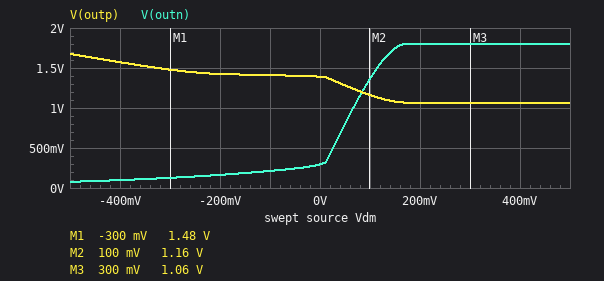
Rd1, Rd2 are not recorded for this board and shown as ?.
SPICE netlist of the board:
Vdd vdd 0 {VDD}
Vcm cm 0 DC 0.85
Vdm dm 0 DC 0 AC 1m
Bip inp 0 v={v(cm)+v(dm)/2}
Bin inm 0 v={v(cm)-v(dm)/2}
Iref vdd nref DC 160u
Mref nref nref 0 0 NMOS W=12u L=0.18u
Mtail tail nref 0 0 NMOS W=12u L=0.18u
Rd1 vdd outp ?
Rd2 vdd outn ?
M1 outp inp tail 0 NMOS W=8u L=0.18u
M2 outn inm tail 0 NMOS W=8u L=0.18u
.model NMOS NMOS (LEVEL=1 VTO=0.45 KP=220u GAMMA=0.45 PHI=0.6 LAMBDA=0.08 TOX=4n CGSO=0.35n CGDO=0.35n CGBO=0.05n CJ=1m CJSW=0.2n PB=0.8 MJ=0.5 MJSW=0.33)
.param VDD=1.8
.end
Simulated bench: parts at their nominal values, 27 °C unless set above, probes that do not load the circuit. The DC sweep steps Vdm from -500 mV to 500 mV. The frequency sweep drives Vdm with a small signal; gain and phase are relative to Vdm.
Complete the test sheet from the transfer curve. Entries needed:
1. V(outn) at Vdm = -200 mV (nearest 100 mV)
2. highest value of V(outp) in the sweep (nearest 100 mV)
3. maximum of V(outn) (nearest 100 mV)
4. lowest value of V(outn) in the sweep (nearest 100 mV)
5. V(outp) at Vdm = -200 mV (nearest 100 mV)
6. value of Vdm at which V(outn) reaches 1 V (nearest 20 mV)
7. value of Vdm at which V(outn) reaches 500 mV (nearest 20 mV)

200 mV
1.7 V
1.8 V
100 mV
1.4 V
60 mV
20 mV
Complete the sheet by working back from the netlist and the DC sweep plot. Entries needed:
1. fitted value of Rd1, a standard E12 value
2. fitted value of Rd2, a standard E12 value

4.7 kΩ
22 kΩ
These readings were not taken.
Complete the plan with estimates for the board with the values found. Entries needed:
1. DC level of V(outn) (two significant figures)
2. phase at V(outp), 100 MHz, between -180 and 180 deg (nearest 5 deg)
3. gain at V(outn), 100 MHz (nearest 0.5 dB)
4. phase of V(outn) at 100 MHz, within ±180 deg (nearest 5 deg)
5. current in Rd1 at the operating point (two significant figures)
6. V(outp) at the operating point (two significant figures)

290 mV
-170 deg
4.5 dB
0 deg
87 µA
1.4 V
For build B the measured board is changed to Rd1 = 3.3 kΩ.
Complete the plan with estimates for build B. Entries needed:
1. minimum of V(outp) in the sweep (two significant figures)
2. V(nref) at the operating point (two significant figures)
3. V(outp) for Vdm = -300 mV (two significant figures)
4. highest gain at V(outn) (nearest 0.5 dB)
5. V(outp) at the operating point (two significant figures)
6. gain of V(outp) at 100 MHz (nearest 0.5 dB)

1.3 V
590 mV
1.6 V
5.0 dB
1.5 V
-11.0 dB
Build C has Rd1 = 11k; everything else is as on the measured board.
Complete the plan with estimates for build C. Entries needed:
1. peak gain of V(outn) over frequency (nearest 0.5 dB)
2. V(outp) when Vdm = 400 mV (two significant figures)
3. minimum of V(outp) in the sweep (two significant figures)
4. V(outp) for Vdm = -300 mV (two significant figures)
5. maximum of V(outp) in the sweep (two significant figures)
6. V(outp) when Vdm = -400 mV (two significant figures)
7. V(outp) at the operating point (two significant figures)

3.5 dB
170 mV
150 mV
1.1 V
1.5 V
1.3 V
850 mV
